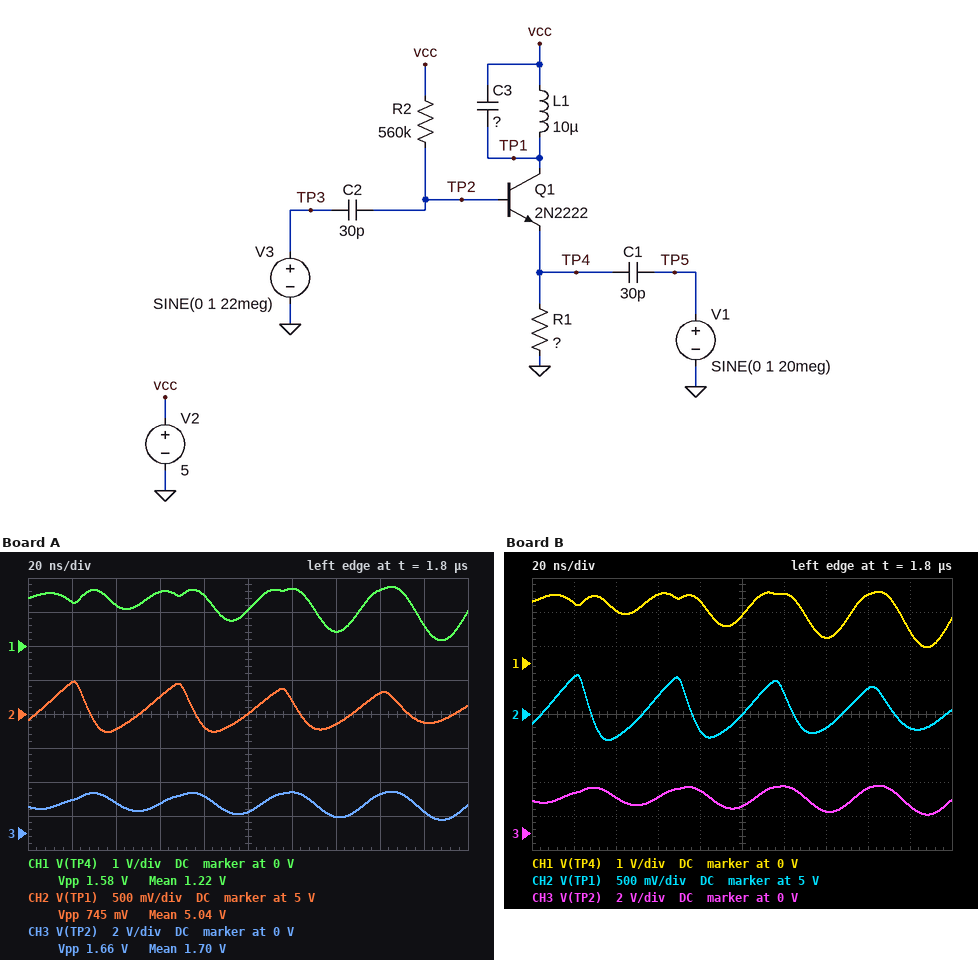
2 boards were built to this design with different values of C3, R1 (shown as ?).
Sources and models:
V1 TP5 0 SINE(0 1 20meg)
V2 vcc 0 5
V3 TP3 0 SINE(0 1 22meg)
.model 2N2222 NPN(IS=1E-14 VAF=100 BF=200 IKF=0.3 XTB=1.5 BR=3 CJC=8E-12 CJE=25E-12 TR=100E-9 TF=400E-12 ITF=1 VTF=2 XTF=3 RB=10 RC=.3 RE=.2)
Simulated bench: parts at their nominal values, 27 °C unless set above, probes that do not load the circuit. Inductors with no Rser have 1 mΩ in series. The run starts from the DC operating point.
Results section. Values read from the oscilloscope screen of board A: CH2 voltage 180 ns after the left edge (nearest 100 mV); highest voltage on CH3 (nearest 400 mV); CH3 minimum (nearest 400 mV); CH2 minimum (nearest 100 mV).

4.9 V
2.4 V
800 mV
4.7 V
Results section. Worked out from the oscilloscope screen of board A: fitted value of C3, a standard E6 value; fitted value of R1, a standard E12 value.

68 pF
820 Ω
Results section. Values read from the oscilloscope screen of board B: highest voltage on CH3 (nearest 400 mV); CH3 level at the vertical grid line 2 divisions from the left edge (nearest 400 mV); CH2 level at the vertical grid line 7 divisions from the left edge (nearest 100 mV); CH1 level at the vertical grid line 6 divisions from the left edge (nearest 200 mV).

2.8 V
2.0 V
4.8 V
2.0 V
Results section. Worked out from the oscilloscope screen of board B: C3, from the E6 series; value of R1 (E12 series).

47 pF
1.2 kΩ
